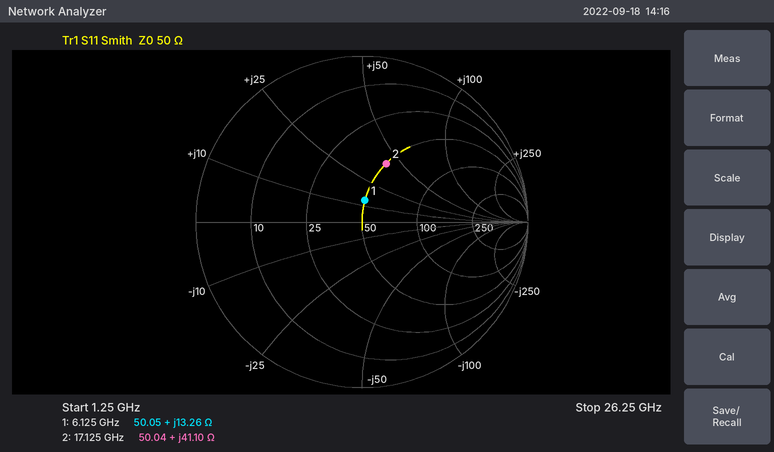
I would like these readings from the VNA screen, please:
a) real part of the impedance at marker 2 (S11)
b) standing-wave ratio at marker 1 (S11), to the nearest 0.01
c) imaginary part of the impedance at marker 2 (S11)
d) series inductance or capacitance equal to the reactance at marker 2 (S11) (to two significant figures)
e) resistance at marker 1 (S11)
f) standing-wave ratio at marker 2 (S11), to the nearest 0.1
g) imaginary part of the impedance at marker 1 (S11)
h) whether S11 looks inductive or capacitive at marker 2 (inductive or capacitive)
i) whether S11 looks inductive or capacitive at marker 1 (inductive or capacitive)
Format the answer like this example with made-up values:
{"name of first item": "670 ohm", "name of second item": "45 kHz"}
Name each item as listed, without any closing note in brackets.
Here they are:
{"real part of the impedance at marker 2": "50.04 Ω", "standing-wave ratio at marker 1 (S11), to the nearest 0.01": "1.30", "imaginary part of the impedance at marker 2": "+41.10 Ω", "series inductance or capacitance equal to the reactance at marker 2 (S11)": "380 pH", "resistance at marker 1": "50.05 Ω", "standing-wave ratio at marker 2 (S11), to the nearest 0.1": "2.2", "imaginary part of the impedance at marker 1": "+13.26 Ω", "whether S11 looks inductive or capacitive at marker 2": "inductive", "whether S11 looks inductive or capacitive at marker 1": "inductive"}
